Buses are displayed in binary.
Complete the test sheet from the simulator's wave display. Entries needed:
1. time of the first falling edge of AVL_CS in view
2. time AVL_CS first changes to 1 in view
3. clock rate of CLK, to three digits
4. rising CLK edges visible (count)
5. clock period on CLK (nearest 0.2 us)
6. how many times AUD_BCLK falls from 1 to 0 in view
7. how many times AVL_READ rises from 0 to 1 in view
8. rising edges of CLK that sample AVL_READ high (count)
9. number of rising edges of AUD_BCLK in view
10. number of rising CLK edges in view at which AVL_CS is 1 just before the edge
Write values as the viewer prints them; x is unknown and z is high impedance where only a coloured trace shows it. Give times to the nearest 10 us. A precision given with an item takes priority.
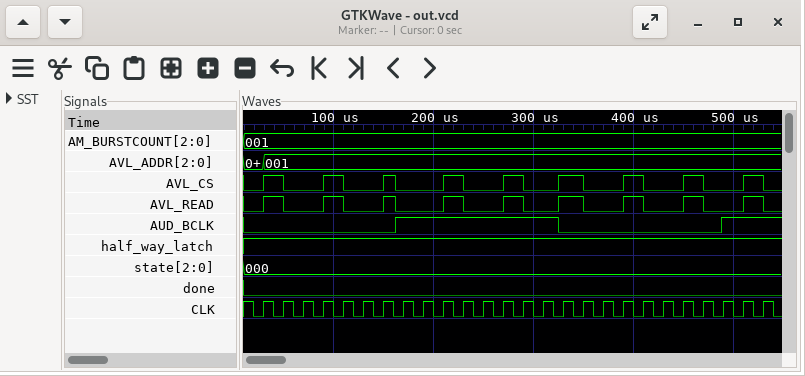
50 us
30 us
50.0 kHz
26
20 us
1
9
9
2
9
